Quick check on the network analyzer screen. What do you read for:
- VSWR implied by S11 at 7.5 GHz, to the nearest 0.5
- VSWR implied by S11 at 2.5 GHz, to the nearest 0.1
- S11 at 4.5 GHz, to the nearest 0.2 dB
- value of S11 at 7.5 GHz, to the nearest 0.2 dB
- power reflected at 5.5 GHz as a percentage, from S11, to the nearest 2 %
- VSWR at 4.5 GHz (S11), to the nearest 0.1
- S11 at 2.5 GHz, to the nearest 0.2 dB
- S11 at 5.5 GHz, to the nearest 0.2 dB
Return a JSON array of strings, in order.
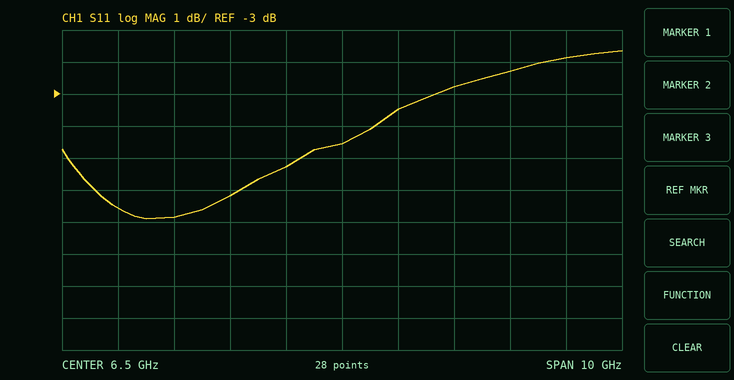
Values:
["5.0", "2.8", "-6.2 dB", "-3.4 dB", "30 %", "2.9", "-6.6 dB", "-5.2 dB"]
